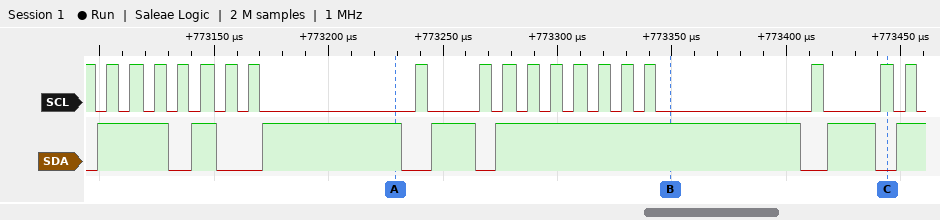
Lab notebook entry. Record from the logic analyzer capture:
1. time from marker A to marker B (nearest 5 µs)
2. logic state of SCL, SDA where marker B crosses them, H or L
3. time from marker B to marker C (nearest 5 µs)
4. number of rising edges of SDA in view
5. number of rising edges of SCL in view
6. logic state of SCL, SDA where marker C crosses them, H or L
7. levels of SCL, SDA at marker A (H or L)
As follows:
120 µs
SCL=L, SDA=H
95 µs
7
19
SCL=H, SDA=L
SCL=L, SDA=H
